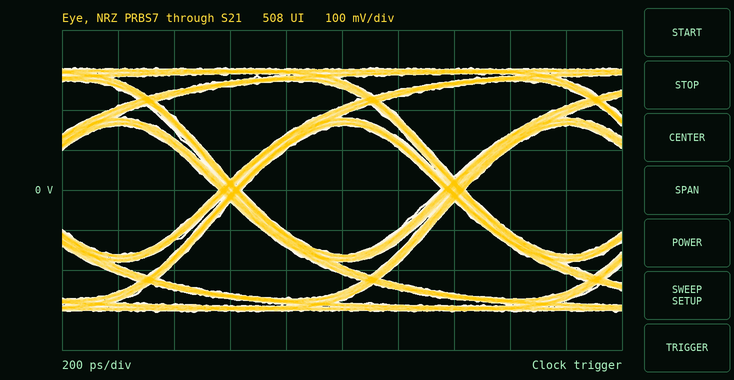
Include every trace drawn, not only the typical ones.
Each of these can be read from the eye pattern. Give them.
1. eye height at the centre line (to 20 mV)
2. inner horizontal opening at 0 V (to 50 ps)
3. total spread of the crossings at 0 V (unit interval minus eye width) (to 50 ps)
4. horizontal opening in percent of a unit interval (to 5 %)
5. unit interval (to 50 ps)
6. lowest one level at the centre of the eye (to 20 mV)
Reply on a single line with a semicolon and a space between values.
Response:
320 mV; 700 ps; 100 ps; 90 %; 800 ps; 160 mV
